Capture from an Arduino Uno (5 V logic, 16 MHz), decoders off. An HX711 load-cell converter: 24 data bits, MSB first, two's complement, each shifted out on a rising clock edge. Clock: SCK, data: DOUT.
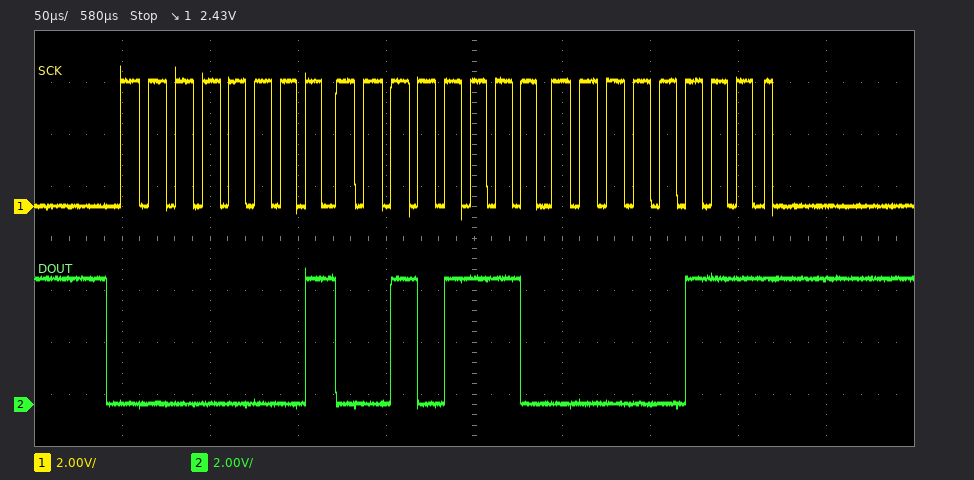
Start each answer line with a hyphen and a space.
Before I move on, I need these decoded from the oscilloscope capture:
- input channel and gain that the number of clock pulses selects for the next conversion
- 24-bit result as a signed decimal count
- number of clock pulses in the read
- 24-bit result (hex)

- channel A, gain 128
- 77319
- 25
- 0x012E07
